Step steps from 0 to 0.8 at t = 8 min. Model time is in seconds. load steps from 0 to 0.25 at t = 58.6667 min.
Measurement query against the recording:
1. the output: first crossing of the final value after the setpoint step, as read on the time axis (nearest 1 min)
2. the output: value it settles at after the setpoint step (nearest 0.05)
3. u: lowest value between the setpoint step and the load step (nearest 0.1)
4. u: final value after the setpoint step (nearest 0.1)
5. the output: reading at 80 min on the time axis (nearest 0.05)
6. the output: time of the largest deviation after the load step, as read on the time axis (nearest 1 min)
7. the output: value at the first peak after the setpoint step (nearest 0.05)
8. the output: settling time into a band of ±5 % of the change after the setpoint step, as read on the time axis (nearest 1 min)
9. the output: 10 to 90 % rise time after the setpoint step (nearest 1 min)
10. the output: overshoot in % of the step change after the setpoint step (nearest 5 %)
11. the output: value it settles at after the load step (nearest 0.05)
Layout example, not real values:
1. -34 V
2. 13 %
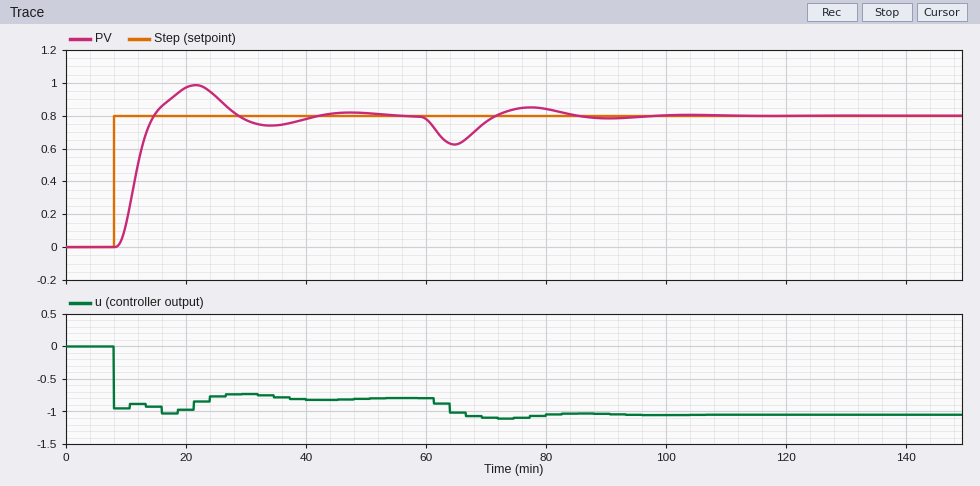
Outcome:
1. 15 min
2. 0.80
3. -1.0
4. -0.8
5. 0.85
6. 65 min
7. 1.00
8. 38 min
9. 4 min
10. 25 %
11. 0.80
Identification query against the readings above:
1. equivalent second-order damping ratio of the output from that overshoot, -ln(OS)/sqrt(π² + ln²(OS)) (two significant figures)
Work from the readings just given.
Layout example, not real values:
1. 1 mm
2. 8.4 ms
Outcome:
1. 0.40
